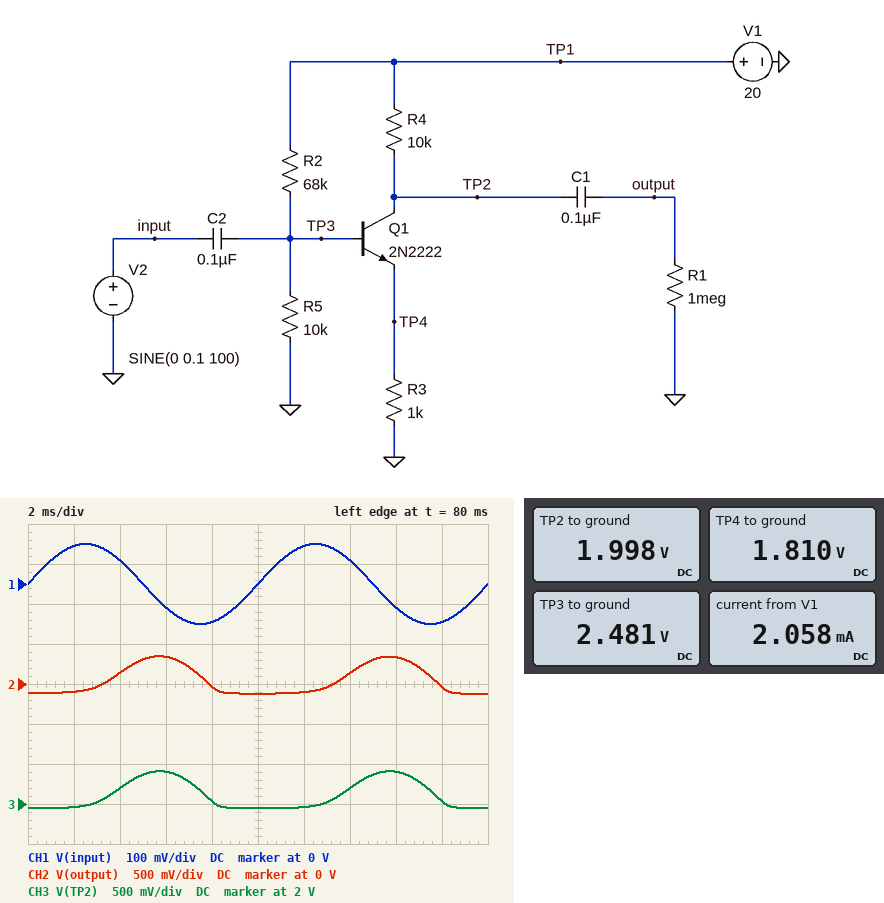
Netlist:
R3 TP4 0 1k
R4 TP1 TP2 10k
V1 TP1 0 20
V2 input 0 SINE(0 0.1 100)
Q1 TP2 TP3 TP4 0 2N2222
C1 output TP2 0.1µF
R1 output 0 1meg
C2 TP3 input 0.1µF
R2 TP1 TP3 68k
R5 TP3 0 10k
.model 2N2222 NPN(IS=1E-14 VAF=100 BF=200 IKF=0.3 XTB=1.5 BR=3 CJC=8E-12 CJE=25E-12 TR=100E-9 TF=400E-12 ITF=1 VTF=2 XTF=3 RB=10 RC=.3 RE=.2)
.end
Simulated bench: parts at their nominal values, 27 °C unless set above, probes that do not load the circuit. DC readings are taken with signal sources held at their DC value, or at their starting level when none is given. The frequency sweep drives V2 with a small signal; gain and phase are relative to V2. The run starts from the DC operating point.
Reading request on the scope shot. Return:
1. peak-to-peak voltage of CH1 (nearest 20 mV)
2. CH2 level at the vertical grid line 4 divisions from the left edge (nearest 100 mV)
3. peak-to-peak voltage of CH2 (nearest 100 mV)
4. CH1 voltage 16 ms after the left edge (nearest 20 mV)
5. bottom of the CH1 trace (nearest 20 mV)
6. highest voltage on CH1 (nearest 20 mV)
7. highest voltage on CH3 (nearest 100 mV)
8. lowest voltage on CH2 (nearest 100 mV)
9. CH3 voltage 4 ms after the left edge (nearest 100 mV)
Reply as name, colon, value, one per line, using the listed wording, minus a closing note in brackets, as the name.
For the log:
peak-to-peak voltage of CH1: 200 mV
CH2 level at the vertical grid line 4 divisions from the left edge: 0 V
peak-to-peak voltage of CH2: 500 mV
CH1 voltage 16 ms after the left edge: -60 mV
bottom of the CH1 trace: -100 mV
highest voltage on CH1: 100 mV
highest voltage on CH3: 2.4 V
lowest voltage on CH2: -100 mV
CH3 voltage 4 ms after the left edge: 2.2 V
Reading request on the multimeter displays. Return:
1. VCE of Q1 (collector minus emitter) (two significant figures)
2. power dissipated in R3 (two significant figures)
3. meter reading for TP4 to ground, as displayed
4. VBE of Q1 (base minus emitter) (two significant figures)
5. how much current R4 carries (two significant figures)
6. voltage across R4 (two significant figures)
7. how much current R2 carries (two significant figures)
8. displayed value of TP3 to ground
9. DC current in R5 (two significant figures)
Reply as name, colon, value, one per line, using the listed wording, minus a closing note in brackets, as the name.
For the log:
VCE of Q1 (collector minus emitter): 190 mV
power dissipated in R3: 3.3 mW
meter reading for TP4 to ground, as displayed: 1.810 V
VBE of Q1 (base minus emitter): 670 mV
how much current R4 carries: 1.8 mA
voltage across R4: 18 V
how much current R2 carries: 260 µA
displayed value of TP3 to ground: 2.481 V
DC current in R5: 250 µA
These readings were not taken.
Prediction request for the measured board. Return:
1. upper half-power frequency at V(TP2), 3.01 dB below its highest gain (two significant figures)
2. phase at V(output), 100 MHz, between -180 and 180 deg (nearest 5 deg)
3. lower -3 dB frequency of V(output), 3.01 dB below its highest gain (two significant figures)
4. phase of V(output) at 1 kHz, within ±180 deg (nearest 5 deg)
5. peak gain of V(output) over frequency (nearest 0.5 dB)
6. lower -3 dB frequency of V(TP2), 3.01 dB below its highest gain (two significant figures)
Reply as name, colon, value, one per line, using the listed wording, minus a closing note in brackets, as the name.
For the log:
upper half-power frequency at V(TP2), 3.01 dB below its highest gain: 1.2 MHz
phase at V(output), 100 MHz, between -180 and 180 deg: 5 deg
lower -3 dB frequency of V(output), 3.01 dB below its highest gain: 440 Hz
phase of V(output) at 1 kHz, within ±180 deg: -155 deg
peak gain of V(output) over frequency: 18.0 dB
lower -3 dB frequency of V(TP2), 3.01 dB below its highest gain: 440 Hz
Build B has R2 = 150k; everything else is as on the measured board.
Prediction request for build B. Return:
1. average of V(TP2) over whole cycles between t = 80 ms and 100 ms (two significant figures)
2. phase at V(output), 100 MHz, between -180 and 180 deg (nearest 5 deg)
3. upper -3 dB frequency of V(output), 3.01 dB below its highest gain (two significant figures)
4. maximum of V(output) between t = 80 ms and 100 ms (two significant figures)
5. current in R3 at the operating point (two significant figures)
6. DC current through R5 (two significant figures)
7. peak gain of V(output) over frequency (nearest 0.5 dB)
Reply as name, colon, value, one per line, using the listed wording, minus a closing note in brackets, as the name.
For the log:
average of V(TP2) over whole cycles between t = 80 ms and 100 ms: 14 V
phase at V(output), 100 MHz, between -180 and 180 deg: 10 deg
upper -3 dB frequency of V(output), 3.01 dB below its highest gain: 5.3 MHz
maximum of V(output) between t = 80 ms and 100 ms: 460 mV
current in R3 at the operating point: 590 µA
DC current through R5: 120 µA
peak gain of V(output) over frequency: 19.5 dB
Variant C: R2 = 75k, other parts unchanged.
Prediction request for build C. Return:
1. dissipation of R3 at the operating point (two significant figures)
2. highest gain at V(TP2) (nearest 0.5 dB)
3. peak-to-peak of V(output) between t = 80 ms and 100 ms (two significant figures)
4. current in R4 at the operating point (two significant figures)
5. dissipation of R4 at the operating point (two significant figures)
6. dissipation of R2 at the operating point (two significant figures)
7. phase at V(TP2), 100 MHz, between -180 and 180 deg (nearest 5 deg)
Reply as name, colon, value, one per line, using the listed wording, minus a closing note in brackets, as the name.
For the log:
dissipation of R3 at the operating point: 2.6 mW
highest gain at V(TP2): 19.5 dB
peak-to-peak of V(output) between t = 80 ms and 100 ms: 900 mV
current in R4 at the operating point: 1.6 mA
dissipation of R4 at the operating point: 26 mW
dissipation of R2 at the operating point: 4.2 mW
phase at V(TP2), 100 MHz, between -180 and 180 deg: 10 deg
